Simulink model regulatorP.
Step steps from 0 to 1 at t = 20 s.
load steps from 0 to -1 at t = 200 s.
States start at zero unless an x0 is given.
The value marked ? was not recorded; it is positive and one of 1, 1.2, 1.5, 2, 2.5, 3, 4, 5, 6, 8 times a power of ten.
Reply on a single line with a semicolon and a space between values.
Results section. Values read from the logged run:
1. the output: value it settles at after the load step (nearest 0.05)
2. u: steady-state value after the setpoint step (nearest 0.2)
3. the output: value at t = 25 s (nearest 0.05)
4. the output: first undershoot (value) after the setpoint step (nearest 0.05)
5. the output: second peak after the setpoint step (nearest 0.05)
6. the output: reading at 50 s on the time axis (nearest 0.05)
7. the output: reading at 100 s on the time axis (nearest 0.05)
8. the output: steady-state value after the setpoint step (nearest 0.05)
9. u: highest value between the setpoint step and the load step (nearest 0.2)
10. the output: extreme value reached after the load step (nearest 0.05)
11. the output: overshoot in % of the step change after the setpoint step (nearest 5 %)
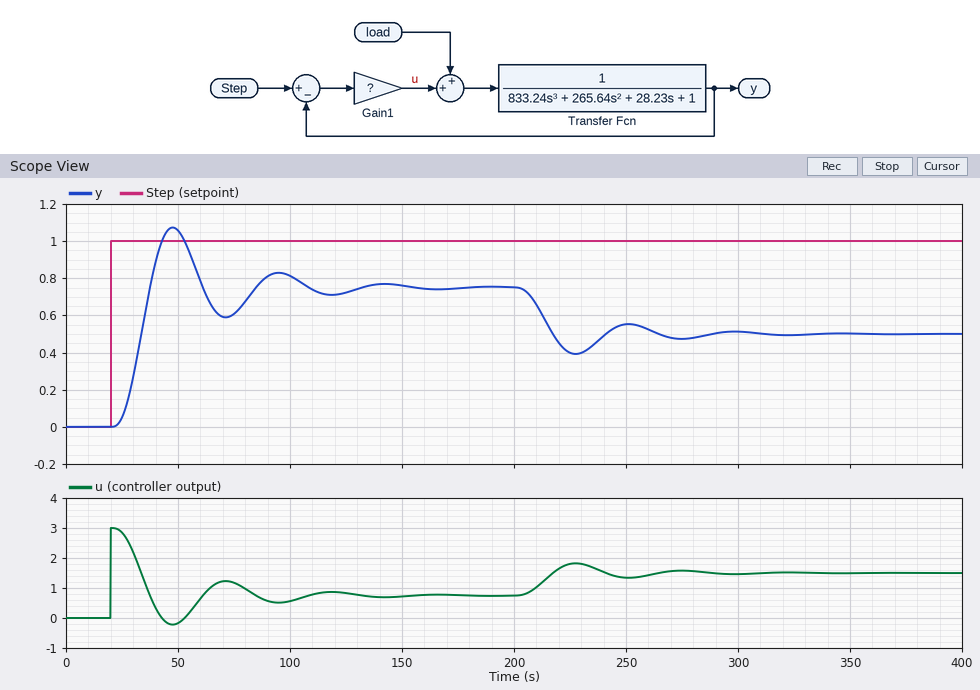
0.50; 0.8; 0.05; 0.60; 0.85; 1.05; 0.80; 0.75; 3.0; 0.40; 45 %
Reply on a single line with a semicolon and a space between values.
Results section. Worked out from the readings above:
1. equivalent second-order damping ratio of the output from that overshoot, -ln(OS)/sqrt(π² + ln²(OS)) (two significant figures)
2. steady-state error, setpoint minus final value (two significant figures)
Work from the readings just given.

0.25; 0.25
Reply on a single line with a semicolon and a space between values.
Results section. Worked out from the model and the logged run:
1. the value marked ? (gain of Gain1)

3
